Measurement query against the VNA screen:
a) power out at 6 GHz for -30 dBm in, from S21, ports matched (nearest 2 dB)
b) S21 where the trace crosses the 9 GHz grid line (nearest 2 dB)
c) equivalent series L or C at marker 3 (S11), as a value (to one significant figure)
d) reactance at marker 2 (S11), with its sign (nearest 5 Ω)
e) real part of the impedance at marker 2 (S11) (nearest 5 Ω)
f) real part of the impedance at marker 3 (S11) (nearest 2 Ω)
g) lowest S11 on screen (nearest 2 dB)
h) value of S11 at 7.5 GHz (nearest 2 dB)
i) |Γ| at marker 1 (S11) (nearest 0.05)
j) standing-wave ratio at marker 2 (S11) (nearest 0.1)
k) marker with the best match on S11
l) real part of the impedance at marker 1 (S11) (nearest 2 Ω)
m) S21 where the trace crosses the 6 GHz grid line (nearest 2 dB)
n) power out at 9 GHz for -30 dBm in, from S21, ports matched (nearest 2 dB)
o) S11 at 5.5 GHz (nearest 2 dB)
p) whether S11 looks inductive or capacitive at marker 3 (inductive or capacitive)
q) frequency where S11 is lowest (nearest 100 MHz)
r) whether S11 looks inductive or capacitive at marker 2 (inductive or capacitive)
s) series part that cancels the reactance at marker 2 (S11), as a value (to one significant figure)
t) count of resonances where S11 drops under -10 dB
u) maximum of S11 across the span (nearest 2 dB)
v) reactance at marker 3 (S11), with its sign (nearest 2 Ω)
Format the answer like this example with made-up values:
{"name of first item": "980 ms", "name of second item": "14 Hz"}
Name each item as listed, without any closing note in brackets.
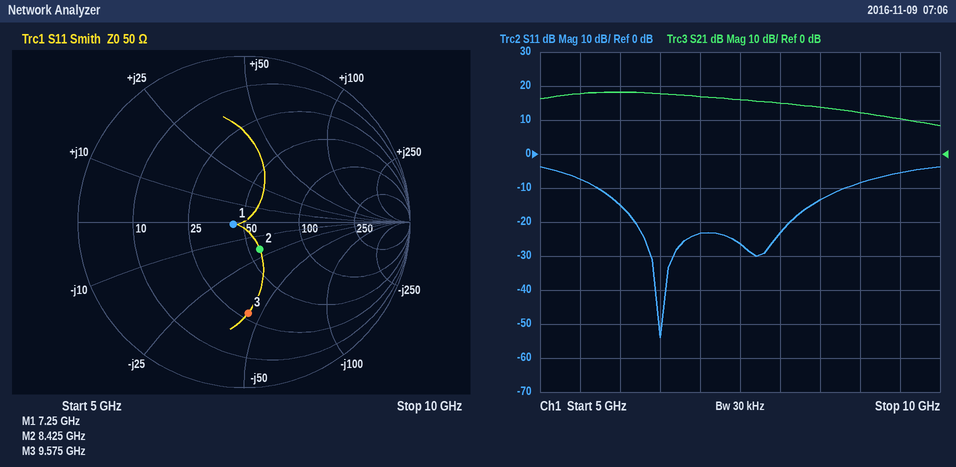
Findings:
{"power out at 6 GHz for -30 dBm in, from S21, ports matched": "-12 dBm", "S21 where the trace crosses the 9 GHz grid line": "12 dB", "equivalent series L or C at marker 3 (S11), as a value": "400 fF", "reactance at marker 2 (S11), with its sign": "-20 Ω", "real part of the impedance at marker 2 (S11)": "55 Ω", "real part of the impedance at marker 3 (S11)": "28 Ω", "lowest S11 on screen": "-54 dB", "value of S11 at 7.5 GHz": "-26 dB", "|Γ| at marker 1 (S11)": "0.05", "standing-wave ratio at marker 2 (S11)": "1.5", "marker with the best match on S11": "marker 1", "real part of the impedance at marker 1 (S11)": "44 Ω", "S21 where the trace crosses the 6 GHz grid line": "18 dB", "power out at 9 GHz for -30 dBm in, from S21, ports matched": "-18 dBm", "S11 at 5.5 GHz": "-8 dB", "whether S11 looks inductive or capacitive at marker 3": "capacitive", "frequency where S11 is lowest": "6.5 GHz", "whether S11 looks inductive or capacitive at marker 2": "capacitive", "series part that cancels the reactance at marker 2 (S11), as a value": "400 pH", "count of resonances where S11 drops under -10 dB": "2", "maximum of S11 across the span": "-4 dB", "reactance at marker 3 (S11), with its sign": "-44 Ω"}
